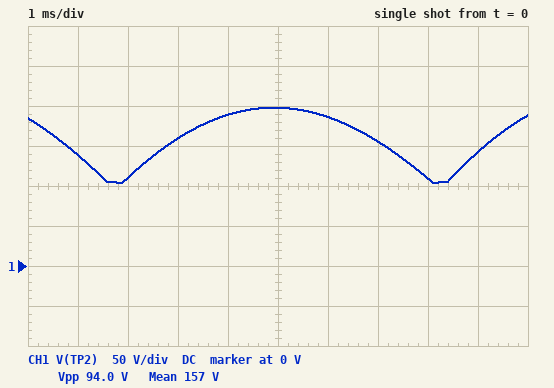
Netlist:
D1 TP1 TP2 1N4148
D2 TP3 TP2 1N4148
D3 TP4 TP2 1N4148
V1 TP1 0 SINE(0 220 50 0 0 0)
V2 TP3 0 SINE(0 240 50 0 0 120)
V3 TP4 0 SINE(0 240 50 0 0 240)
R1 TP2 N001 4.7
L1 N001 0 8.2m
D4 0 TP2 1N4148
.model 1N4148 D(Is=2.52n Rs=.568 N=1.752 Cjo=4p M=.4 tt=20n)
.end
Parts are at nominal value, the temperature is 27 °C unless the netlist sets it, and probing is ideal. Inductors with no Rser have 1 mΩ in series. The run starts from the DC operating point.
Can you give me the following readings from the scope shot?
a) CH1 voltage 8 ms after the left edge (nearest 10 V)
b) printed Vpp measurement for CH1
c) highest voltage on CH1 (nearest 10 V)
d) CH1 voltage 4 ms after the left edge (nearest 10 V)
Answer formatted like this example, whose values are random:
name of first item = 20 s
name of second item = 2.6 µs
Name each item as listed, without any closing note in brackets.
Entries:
CH1 voltage 8 ms after the left edge = 110 V
printed Vpp measurement for CH1 = 94.0 V
highest voltage on CH1 = 200 V
CH1 voltage 4 ms after the left edge = 190 V
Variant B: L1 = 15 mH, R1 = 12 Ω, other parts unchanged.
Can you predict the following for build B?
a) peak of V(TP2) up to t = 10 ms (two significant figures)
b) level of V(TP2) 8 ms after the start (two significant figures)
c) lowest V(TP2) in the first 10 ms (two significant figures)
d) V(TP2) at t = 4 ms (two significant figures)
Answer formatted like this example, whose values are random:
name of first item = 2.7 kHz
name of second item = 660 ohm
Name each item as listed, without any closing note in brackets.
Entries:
peak of V(TP2) up to t = 10 ms = 210 V
level of V(TP2) 8 ms after the start = 120 V
lowest V(TP2) in the first 10 ms = 110 V
V(TP2) at t = 4 ms = 200 V
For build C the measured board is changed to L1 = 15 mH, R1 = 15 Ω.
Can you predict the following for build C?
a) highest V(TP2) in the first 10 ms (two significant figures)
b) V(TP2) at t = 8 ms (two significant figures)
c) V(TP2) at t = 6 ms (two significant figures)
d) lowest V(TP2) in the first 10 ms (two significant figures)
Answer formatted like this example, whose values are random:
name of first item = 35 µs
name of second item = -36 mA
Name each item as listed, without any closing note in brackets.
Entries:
highest V(TP2) in the first 10 ms = 210 V
V(TP2) at t = 8 ms = 120 V
V(TP2) at t = 6 ms = 200 V
lowest V(TP2) in the first 10 ms = 110 V
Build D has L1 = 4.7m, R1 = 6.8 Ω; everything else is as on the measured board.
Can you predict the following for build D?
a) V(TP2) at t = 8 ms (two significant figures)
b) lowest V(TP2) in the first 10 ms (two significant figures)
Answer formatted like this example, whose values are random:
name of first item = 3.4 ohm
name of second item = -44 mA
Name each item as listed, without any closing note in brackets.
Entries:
V(TP2) at t = 8 ms = 120 V
lowest V(TP2) in the first 10 ms = 110 V
